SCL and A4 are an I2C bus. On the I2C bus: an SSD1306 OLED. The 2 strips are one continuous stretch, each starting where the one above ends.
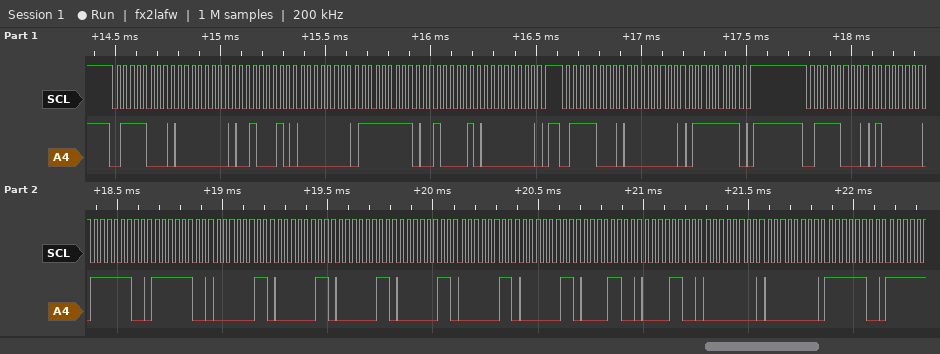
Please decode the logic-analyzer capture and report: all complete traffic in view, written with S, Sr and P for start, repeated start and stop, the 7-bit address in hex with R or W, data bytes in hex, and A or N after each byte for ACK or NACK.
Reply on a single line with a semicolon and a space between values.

S 3CW A 00 A 22 A 00 A FF A 21 A 00 A P S 3CW A 00 A 7F A P S 3CW A 40 A FC A FC A 03 A 03 A 03 A 03 A 03 A 03 A 0C A 0C A 00 A 00 A FC A
